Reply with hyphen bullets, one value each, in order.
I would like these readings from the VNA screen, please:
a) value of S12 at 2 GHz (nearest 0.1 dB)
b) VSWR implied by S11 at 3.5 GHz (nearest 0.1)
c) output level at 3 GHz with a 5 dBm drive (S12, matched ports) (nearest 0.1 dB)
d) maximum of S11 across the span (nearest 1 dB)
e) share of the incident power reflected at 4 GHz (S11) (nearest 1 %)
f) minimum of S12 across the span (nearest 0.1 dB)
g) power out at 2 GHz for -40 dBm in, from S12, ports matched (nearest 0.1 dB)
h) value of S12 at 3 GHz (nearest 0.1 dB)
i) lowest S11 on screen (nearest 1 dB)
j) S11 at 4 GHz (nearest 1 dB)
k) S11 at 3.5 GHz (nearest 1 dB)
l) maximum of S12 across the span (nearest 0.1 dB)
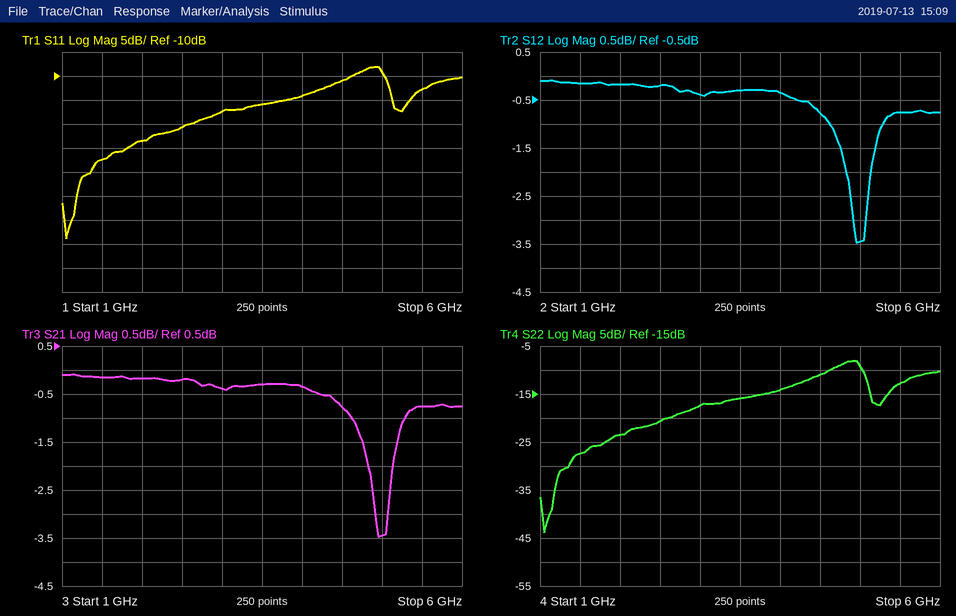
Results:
- -0.2 dB
- 1.4
- 4.6 dBm
- -8 dB
- 4 %
- -3.5 dB
- -40.2 dBm
- -0.4 dB
- -44 dB
- -14 dB
- -16 dB
- -0.1 dB
